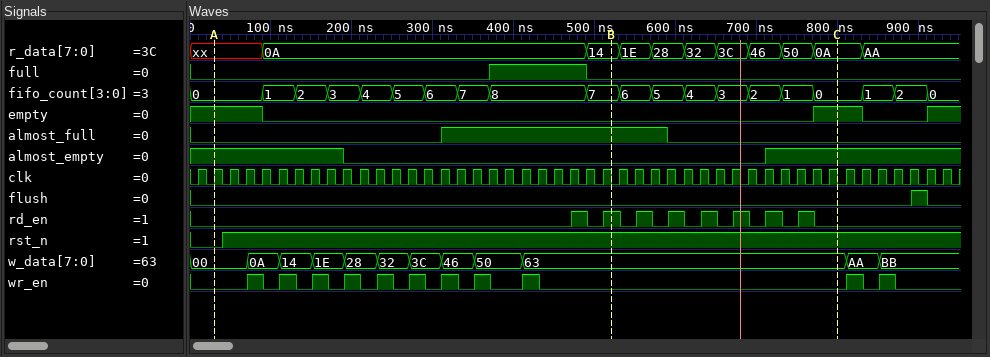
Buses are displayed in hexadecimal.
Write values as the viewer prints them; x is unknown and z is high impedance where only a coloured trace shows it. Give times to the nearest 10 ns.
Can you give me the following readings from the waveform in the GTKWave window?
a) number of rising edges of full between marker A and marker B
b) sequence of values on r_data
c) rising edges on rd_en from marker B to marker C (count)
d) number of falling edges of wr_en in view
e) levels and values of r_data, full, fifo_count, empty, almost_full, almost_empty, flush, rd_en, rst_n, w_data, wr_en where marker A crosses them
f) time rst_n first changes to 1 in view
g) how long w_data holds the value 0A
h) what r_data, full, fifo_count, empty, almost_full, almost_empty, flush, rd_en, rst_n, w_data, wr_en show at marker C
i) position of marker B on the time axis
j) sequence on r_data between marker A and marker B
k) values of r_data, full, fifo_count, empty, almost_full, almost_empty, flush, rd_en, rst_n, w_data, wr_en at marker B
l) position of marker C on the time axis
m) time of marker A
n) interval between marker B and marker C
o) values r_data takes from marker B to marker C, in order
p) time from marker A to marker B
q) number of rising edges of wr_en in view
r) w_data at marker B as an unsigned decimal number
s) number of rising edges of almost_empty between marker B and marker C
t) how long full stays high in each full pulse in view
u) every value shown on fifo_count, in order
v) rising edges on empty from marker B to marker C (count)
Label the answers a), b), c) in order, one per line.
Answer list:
a) 1
b) xx, 0A, 14, 1E, 28, 32, 3C, 46, 50, 0A, AA
c) 6
d) 11
e) r_data=xx, full=0, fifo_count=0, empty=1, almost_full=0, almost_empty=1, flush=0, rd_en=0, rst_n=0, w_data=00, wr_en=0
f) 40 ns
g) 40 ns
h) r_data=0A, full=0, fifo_count=0, empty=1, almost_full=0, almost_empty=1, flush=0, rd_en=0, rst_n=1, w_data=63, wr_en=0
i) 520 ns
j) xx, 0A, 14
k) r_data=14, full=0, fifo_count=7, empty=0, almost_full=1, almost_empty=0, flush=0, rd_en=1, rst_n=1, w_data=63, wr_en=0
l) 800 ns
m) 30 ns
n) 280 ns
o) 14, 1E, 28, 32, 3C, 46, 50, 0A
p) 490 ns
q) 11
r) 99
s) 1
t) 120 ns
u) 0, 1, 2, 3, 4, 5, 6, 7, 8, 7, 6, 5, 4, 3, 2, 1, 0, 1, 2, 0
v) 1
